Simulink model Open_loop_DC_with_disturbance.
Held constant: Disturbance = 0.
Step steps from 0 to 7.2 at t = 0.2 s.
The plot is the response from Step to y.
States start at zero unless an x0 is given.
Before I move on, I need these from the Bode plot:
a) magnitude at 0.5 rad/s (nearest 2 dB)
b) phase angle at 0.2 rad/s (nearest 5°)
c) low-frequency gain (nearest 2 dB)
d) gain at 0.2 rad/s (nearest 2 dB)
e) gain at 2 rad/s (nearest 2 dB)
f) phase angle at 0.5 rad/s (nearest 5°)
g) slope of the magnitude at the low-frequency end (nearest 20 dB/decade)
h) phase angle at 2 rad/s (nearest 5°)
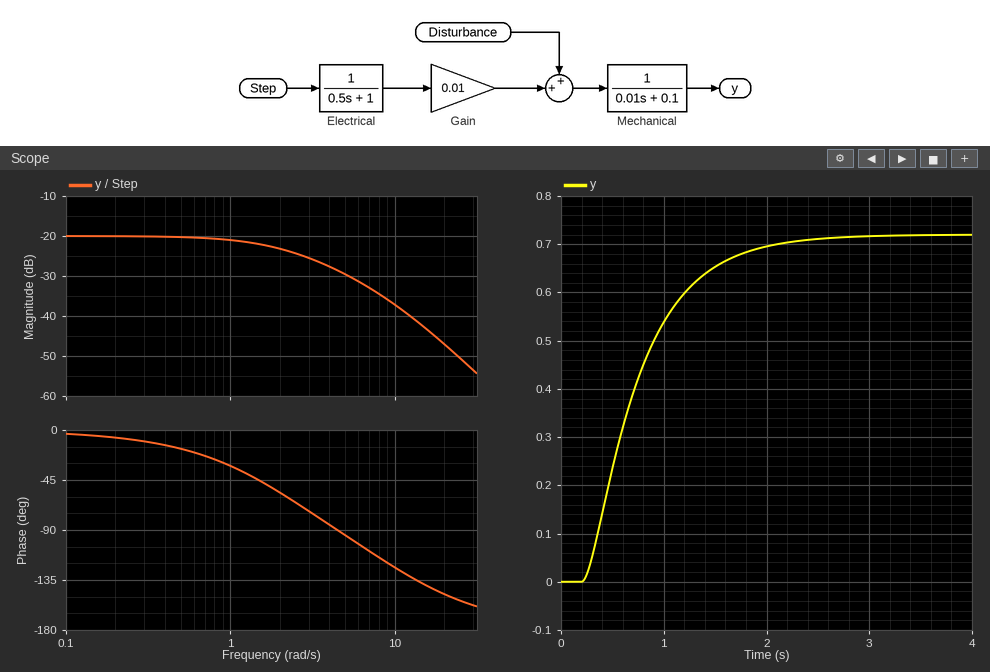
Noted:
-20 dB
-5°
-20 dB
-20 dB
-24 dB
-15°
0 dB/decade
-55°
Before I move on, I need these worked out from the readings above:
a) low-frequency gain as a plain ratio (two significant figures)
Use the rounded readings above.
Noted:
0.10
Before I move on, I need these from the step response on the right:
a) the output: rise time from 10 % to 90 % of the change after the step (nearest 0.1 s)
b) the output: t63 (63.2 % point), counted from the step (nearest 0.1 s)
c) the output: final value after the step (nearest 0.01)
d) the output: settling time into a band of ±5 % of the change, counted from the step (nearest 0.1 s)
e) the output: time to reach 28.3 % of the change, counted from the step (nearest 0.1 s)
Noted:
1.1 s
0.6 s
0.72
1.6 s
0.3 s
